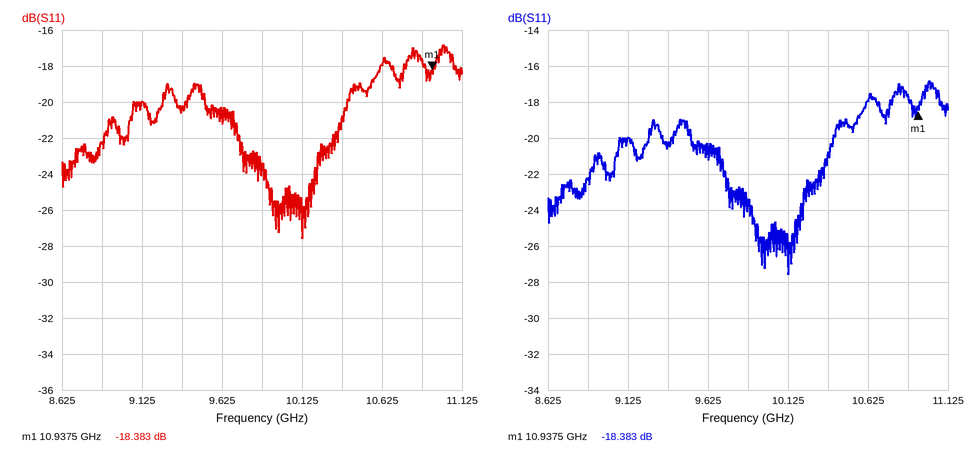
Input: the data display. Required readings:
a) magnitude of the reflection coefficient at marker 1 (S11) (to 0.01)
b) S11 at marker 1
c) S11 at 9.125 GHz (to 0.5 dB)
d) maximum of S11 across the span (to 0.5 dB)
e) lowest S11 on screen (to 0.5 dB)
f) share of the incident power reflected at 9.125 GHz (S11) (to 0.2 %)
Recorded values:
0.12
-18.383 dB
-20.0 dB
-17.0 dB
-27.5 dB
1.0 %
